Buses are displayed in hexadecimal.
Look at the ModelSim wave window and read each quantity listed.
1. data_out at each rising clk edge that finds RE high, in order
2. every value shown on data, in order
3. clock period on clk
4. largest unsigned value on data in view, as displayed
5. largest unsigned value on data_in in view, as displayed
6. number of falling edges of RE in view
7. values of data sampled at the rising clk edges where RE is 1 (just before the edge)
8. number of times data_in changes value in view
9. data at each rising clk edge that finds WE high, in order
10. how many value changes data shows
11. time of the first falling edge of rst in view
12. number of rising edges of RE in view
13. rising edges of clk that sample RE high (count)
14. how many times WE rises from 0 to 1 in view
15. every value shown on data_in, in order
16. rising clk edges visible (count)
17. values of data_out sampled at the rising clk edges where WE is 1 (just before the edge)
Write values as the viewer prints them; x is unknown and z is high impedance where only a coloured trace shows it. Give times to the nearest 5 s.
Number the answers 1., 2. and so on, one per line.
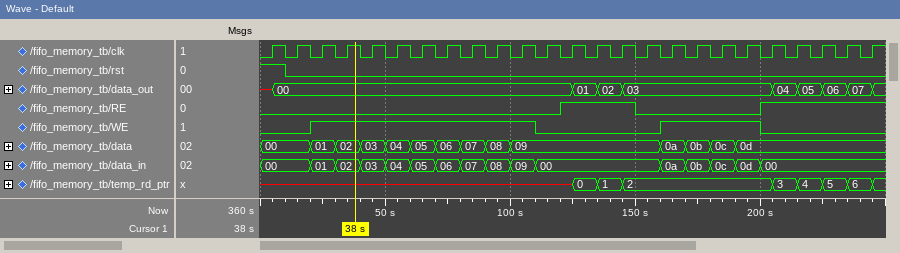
1. 00, 01, 02, 03, 04, 05, 06, 07
2. 00, 01, 02, 03, 04, 05, 06, 07, 08, 09, 0a, 0b, 0c, 0d
3. 10 s
4. 0d
5. 0d
6. 1
7. 09, 09, 09, 0d, 0d, 0d, 0d, 0d
8. 15
9. 01, 02, 03, 04, 05, 06, 07, 08, 09, 0a, 0b, 0c, 0d
10. 13
11. 10 s
12. 2
13. 8
14. 2
15. 00, 01, 02, 03, 04, 05, 06, 07, 08, 09, 00, 0a, 0b, 0c, 0d, 00
16. 25
17. 00, 00, 00, 00, 00, 00, 00, 00, 00, 03, 03, 03, 03
